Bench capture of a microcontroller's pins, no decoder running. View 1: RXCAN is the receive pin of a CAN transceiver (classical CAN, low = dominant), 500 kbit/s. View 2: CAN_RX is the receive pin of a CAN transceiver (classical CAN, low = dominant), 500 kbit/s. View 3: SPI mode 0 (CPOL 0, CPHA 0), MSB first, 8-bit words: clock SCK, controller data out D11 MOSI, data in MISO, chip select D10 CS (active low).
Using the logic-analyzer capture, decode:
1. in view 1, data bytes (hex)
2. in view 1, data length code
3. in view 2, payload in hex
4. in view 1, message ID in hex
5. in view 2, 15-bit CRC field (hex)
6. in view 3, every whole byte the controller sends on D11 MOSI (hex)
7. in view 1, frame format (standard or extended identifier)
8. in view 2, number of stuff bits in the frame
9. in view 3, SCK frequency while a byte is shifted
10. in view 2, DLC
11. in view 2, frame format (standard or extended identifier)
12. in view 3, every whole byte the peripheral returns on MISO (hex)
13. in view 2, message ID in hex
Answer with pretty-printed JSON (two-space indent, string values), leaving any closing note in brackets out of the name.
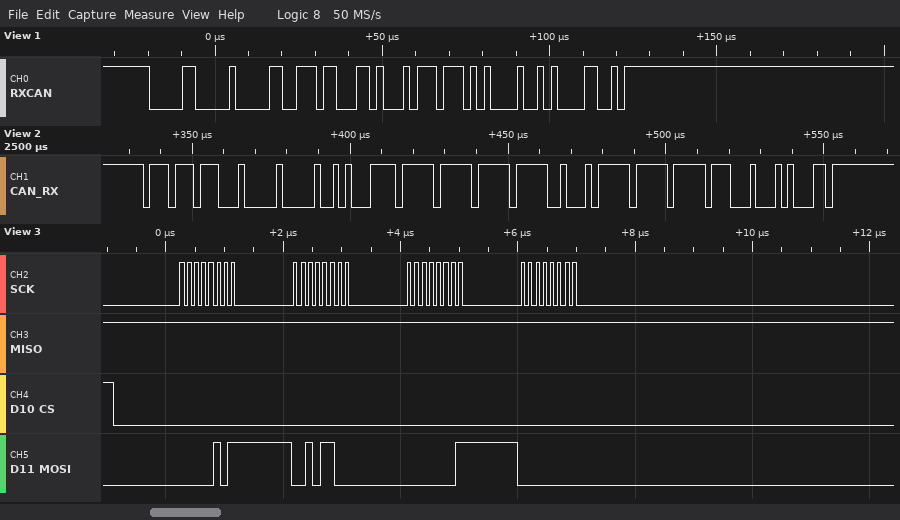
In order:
{
  "in view 1, data bytes": "EC 68 BB A8",
  "in view 1, data length code": "4",
  "in view 2, payload in hex": "00 51 EF FF FF 45 FF FF",
  "in view 1, message ID in hex": "0x040",
  "in view 2, 15-bit CRC field": "0x4451",
  "in view 3, every whole byte the controller sends on D11 MOSI": "0x05 0x2C 0x01 0x00",
  "in view 1, frame format": "standard",
  "in view 2, number of stuff bits in the frame": "9",
  "in view 3, SCK frequency while a byte is shifted": "8 MHz",
  "in view 2, DLC": "8",
  "in view 2, frame format": "standard",
  "in view 3, every whole byte the peripheral returns on MISO": "0xFF 0xFF 0xFF 0xFF",
  "in view 2, message ID in hex": "0x777"
}
